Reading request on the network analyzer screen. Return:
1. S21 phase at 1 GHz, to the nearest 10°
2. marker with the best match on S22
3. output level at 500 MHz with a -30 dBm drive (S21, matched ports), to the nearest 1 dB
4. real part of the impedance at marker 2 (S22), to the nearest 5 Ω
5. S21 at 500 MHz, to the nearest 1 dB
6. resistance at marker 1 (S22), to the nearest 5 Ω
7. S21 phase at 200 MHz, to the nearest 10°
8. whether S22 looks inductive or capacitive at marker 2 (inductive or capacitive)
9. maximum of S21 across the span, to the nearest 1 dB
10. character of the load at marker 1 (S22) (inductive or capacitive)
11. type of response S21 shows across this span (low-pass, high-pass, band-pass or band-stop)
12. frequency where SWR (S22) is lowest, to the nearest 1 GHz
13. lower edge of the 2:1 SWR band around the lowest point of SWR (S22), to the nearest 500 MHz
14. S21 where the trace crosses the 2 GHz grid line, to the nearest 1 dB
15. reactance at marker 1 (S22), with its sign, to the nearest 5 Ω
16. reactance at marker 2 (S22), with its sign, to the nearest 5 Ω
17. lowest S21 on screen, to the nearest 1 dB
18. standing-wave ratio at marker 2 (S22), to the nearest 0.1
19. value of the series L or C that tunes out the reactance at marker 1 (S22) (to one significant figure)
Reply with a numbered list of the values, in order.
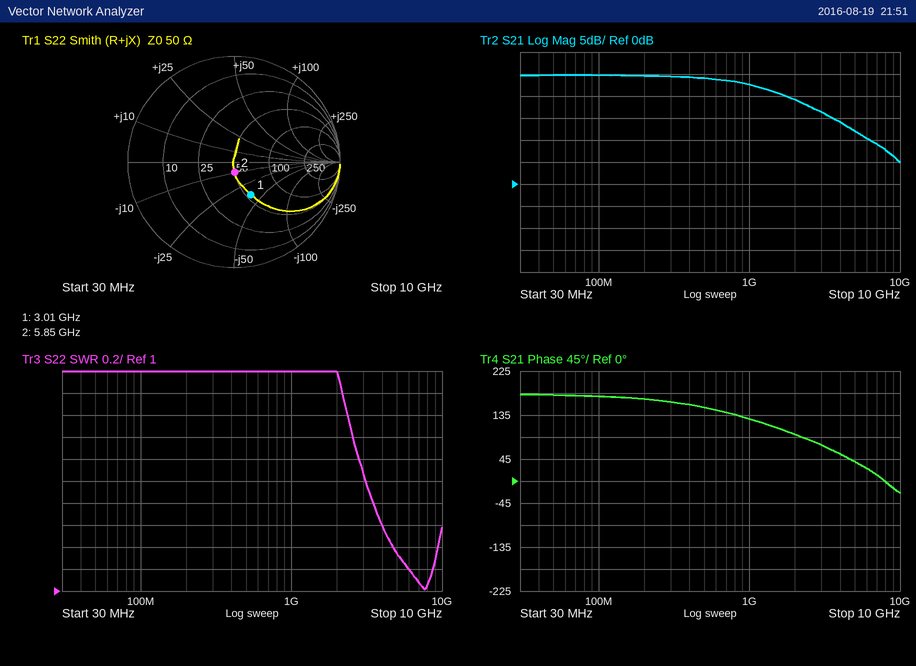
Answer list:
1. 130°
2. marker 2
3. -6 dBm
4. 50 Ω
5. 24 dB
6. 55 Ω
7. 170°
8. capacitive
9. 25 dB
10. capacitive
11. low-pass
12. 8 GHz
13. 3.0 GHz
14. 19 dB
15. -40 Ω
16. -10 Ω
17. 5 dB
18. 1.2
19. 2 nH
